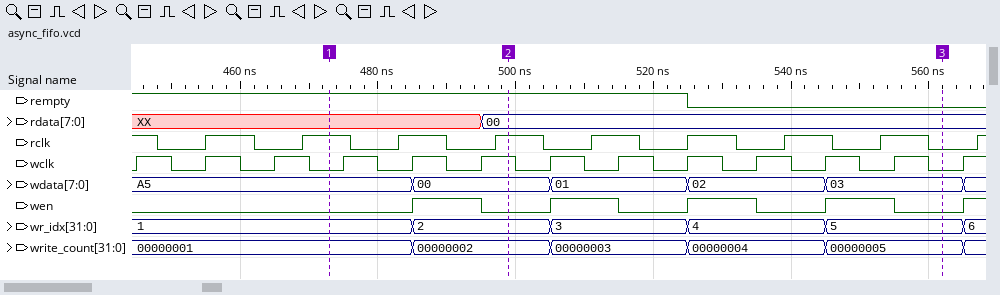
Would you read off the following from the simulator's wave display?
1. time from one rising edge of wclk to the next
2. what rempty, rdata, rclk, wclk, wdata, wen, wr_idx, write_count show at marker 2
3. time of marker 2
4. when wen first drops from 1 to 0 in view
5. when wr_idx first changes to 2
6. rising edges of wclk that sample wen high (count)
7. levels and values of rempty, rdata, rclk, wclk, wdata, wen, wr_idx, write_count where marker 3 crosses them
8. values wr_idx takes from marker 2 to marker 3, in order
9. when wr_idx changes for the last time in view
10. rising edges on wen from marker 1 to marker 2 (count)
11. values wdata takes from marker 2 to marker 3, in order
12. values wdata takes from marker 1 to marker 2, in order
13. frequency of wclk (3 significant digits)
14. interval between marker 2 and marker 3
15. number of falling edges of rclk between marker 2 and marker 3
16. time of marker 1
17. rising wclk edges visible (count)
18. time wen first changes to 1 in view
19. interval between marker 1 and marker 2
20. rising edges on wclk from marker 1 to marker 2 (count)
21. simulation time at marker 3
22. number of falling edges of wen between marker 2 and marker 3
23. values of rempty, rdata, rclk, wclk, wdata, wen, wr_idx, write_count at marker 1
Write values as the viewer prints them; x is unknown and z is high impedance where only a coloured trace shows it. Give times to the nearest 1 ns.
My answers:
10 ns
rempty=1, rdata=00, rclk=1, wclk=1, wdata=00, wen=0, wr_idx=2, write_count=00000002
499 ns
495 ns
485 ns
4
rempty=0, rdata=00, rclk=0, wclk=0, wdata=03, wen=0, wr_idx=5, write_count=00000005
2, 3, 4, 5
565 ns
1
00, 01, 02, 03
A5, 00
100 MHz
63 ns
5
473 ns
13
485 ns
26 ns
3
562 ns
3
rempty=1, rdata=XX, rclk=1, wclk=0, wdata=A5, wen=0, wr_idx=1, write_count=00000001
